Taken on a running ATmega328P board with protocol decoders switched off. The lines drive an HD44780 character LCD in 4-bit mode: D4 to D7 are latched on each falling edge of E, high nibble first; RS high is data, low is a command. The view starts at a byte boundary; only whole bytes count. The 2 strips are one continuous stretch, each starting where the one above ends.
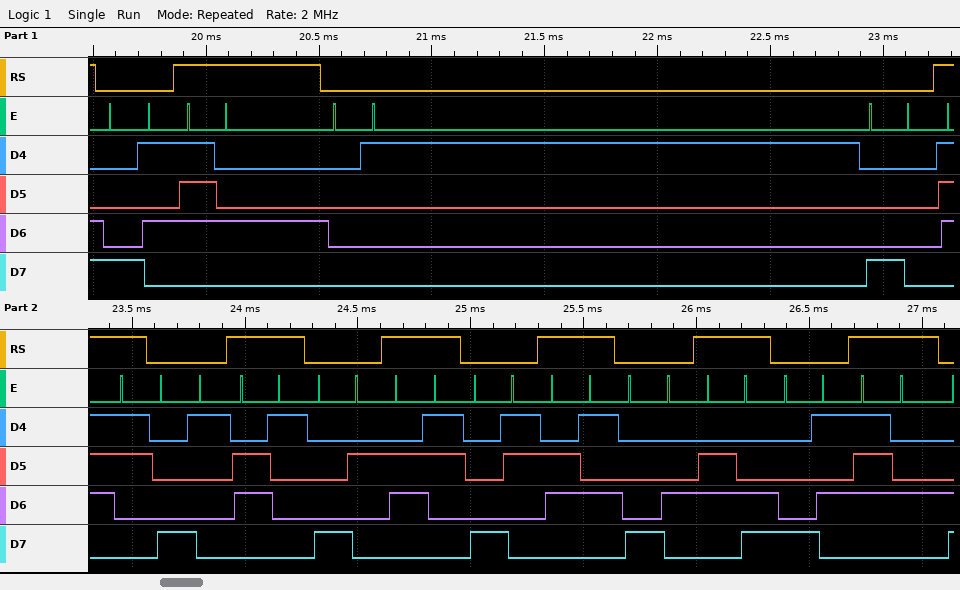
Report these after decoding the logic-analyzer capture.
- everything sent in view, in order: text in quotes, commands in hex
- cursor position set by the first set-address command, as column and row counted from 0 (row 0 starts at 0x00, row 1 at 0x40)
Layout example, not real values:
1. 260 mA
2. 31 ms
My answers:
1. 0x85 "t" 0x01 0x80 "s" 0x81 "a" 0x82 "c" 0x83 "e" 0x84 "l" 0x85 "t"
2. column 5, row 0
